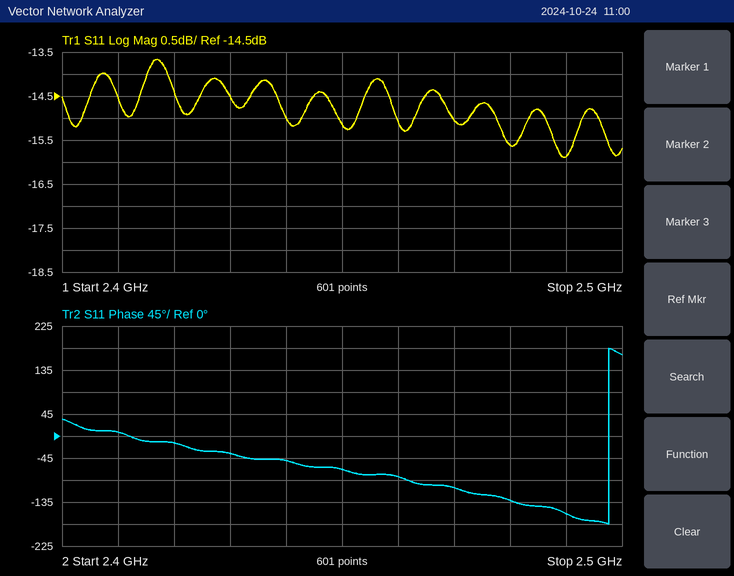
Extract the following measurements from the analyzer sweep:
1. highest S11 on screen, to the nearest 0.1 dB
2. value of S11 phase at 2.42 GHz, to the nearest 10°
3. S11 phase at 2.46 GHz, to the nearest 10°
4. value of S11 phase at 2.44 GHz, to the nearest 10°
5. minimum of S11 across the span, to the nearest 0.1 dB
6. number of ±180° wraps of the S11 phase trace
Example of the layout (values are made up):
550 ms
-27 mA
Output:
-13.7 dB
-10°
-80°
-50°
-15.9 dB
1
